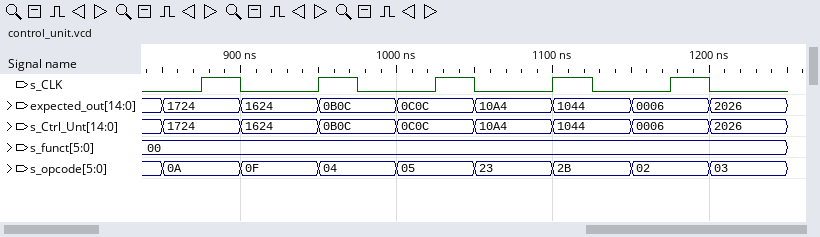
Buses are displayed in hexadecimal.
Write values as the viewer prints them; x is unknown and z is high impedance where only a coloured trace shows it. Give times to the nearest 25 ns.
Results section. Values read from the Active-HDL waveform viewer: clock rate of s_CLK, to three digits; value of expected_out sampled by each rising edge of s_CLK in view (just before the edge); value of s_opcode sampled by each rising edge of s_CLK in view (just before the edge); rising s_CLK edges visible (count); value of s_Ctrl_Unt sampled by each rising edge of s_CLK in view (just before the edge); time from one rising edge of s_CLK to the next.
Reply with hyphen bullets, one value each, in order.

- 13.3 MHz
- 1724, 1624, 0C0C, 10A4, 0006
- 0A, 0F, 05, 23, 02
- 5
- 1724, 1624, 0C0C, 10A4, 0006
- 75 ns
